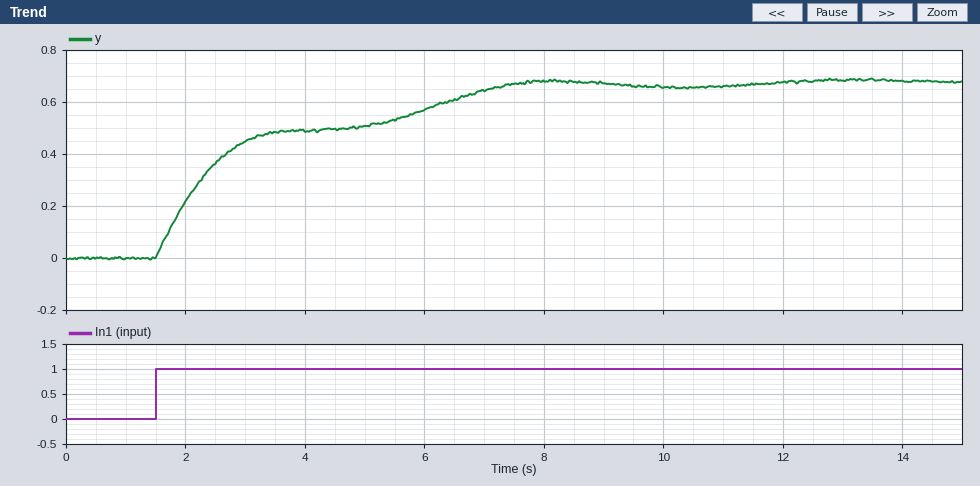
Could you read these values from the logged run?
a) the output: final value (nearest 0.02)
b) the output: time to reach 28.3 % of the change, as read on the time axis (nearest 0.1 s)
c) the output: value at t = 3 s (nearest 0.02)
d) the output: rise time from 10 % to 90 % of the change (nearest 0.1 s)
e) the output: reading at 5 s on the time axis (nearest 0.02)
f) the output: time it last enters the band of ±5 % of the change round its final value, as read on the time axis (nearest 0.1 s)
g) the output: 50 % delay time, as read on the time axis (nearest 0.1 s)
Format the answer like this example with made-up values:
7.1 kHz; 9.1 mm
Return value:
0.68; 1.9 s; 0.44; 4.9 s; 0.50; 7.0 s; 2.4 s
